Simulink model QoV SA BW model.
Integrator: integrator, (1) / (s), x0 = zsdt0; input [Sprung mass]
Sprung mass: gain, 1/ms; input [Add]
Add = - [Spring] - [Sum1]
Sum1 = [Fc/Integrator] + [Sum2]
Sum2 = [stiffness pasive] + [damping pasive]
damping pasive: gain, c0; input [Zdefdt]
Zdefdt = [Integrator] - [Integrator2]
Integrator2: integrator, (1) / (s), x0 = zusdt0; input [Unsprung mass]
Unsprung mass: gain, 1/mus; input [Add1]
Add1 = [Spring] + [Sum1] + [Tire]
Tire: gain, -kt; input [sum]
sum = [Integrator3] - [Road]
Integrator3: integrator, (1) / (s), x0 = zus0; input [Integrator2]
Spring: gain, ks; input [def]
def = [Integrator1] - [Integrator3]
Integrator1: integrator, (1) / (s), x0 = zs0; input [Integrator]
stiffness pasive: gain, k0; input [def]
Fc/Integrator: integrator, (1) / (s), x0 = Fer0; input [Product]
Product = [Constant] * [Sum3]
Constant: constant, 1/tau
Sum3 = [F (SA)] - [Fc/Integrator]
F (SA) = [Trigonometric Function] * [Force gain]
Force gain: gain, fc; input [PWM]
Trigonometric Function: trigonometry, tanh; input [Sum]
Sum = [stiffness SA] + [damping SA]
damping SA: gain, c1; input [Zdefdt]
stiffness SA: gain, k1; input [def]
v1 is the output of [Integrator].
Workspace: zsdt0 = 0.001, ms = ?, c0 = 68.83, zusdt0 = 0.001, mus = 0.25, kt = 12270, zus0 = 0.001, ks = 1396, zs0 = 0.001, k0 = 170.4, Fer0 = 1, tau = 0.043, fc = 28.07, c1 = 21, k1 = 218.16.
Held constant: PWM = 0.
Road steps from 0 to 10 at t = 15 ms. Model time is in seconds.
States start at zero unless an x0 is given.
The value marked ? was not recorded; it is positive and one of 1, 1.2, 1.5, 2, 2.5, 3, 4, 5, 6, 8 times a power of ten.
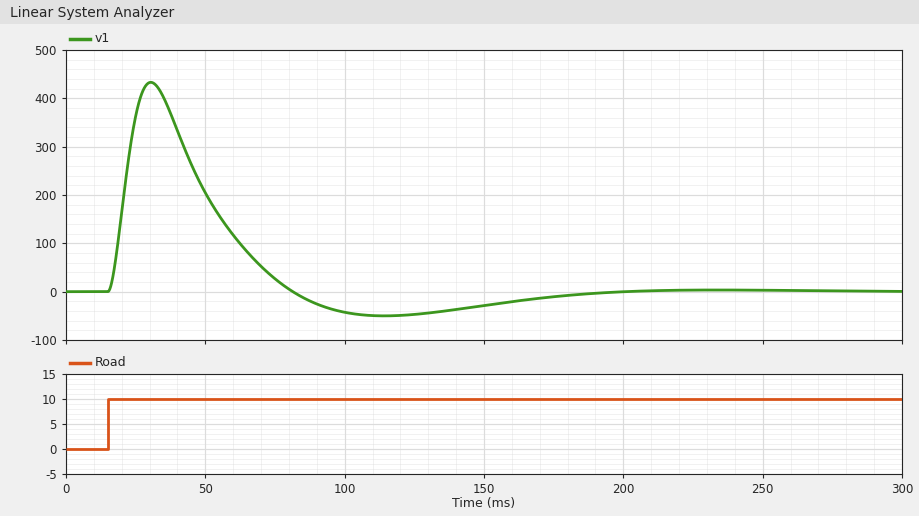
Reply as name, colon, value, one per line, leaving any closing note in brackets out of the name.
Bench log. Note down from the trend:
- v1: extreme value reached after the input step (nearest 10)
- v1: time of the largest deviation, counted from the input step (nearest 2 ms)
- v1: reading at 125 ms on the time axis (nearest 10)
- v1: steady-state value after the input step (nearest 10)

v1: extreme value reached after the input step: 430
v1: time of the largest deviation, counted from the input step: 16 ms
v1: reading at 125 ms on the time axis: -50
v1: steady-state value after the input step: 0
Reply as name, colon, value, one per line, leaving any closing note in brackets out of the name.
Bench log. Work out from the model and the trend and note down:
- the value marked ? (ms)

the value marked ?: 1.5
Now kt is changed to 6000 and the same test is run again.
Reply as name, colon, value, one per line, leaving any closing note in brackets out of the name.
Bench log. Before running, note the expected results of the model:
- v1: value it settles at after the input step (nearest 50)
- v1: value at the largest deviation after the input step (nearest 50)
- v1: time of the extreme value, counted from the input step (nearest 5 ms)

v1: value it settles at after the input step: 0
v1: value at the largest deviation after the input step: 350
v1: time of the extreme value, counted from the input step: 25 ms
